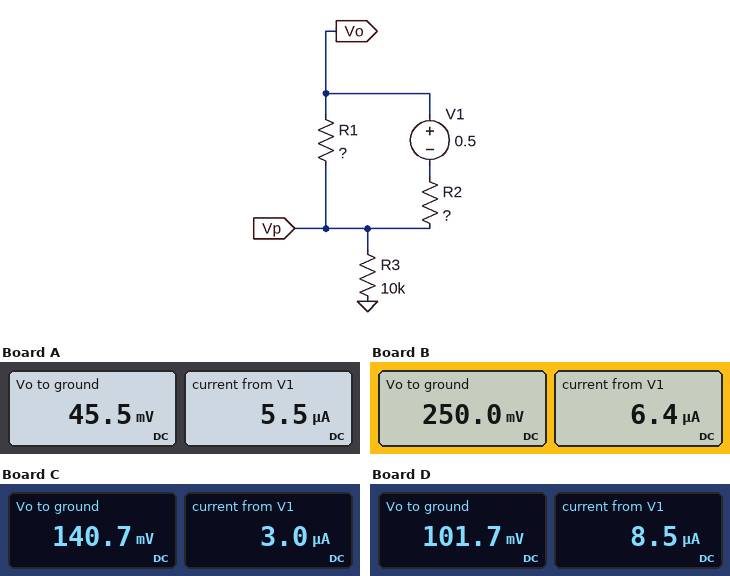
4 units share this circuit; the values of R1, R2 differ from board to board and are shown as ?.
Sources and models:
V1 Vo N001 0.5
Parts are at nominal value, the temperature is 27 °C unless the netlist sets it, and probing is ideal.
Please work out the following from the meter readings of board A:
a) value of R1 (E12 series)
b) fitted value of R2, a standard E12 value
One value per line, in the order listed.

8.2 kΩ
82 kΩ
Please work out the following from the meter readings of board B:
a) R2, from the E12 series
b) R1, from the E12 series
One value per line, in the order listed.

39 kΩ
39 kΩ
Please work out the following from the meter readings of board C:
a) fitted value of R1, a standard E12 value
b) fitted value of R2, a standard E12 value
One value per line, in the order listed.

47 kΩ
120 kΩ
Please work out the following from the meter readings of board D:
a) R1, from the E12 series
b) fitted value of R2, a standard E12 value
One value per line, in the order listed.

12 kΩ
47 kΩ
